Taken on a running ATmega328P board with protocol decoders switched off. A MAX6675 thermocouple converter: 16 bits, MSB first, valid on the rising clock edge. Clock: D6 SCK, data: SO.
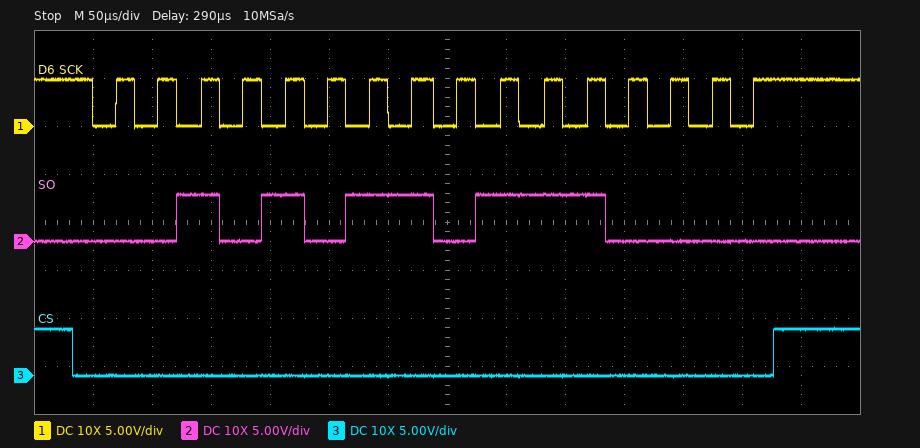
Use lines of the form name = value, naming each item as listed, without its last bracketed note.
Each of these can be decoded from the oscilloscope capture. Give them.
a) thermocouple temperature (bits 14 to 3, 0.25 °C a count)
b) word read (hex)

thermocouple temperature = 347.50 °C
word read = 0x2B70
